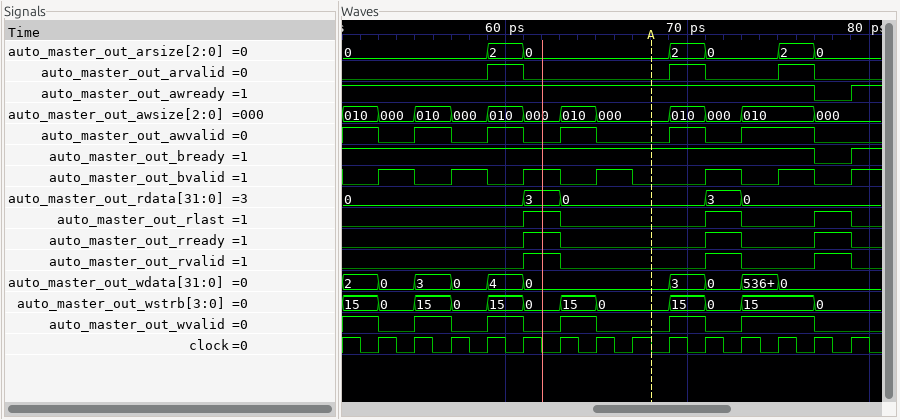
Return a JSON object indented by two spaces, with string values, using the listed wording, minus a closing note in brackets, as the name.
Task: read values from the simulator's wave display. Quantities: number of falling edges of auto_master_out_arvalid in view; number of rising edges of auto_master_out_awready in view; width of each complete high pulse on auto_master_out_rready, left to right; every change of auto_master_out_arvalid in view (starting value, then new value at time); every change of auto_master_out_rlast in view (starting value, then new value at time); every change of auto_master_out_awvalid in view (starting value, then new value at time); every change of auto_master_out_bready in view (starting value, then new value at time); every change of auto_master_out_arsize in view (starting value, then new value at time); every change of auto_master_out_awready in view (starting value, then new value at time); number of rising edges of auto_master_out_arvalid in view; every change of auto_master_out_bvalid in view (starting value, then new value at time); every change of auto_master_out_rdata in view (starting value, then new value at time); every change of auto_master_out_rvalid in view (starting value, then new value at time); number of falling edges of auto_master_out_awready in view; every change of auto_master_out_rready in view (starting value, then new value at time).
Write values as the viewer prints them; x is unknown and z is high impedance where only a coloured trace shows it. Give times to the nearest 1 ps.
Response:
{
  "number of falling edges of auto_master_out_arvalid in view": "3",
  "number of rising edges of auto_master_out_awready in view": "1",
  "width of each complete high pulse on auto_master_out_rready, left to right": "2 ps, 2 ps, 2 ps",
  "every change of auto_master_out_arvalid in view": "0, 1 at 59 ps, 0 at 61 ps, 1 at 69 ps, 0 at 71 ps, 1 at 75 ps, 0 at 77 ps",
  "every change of auto_master_out_rlast in view": "0, 1 at 61 ps, 0 at 63 ps, 1 at 71 ps, 0 at 73 ps, 1 at 77 ps, 0 at 79 ps",
  "every change of auto_master_out_awvalid in view": "1, 0 at 53 ps, 1 at 55 ps, 0 at 57 ps, 1 at 59 ps, 0 at 61 ps, 1 at 63 ps, 0 at 65 ps, 1 at 69 ps, 0 at 71 ps, 1 at 73 ps, 0 at 77 ps",
  "every change of auto_master_out_bready in view": "1, 0 at 77 ps, 1 at 79 ps",
  "every change of auto_master_out_arsize in view": "0, 2 at 59 ps, 0 at 61 ps, 2 at 69 ps, 0 at 71 ps, 2 at 75 ps, 0 at 77 ps",
  "every change of auto_master_out_awready in view": "1, 0 at 77 ps, 1 at 79 ps",
  "number of rising edges of auto_master_out_arvalid in view": "3",
  "every change of auto_master_out_bvalid in view": "0, 1 at 53 ps, 0 at 55 ps, 1 at 57 ps, 0 at 59 ps, 1 at 61 ps, 0 at 63 ps, 1 at 65 ps, 0 at 67 ps, 1 at 71 ps, 0 at 73 ps, 1 at 75 ps, 0 at 77 ps, 1 at 79 ps",
  "every change of auto_master_out_rdata in view": "0, 3 at 61 ps, 0 at 63 ps, 3 at 71 ps, 0 at 73 ps",
  "every change of auto_master_out_rvalid in view": "0, 1 at 61 ps, 0 at 63 ps, 1 at 71 ps, 0 at 73 ps, 1 at 77 ps, 0 at 79 ps",
  "number of falling edges of auto_master_out_awready in view": "1",
  "every change of auto_master_out_rready in view": "0, 1 at 61 ps, 0 at 63 ps, 1 at 71 ps, 0 at 73 ps, 1 at 77 ps, 0 at 79 ps"
}
